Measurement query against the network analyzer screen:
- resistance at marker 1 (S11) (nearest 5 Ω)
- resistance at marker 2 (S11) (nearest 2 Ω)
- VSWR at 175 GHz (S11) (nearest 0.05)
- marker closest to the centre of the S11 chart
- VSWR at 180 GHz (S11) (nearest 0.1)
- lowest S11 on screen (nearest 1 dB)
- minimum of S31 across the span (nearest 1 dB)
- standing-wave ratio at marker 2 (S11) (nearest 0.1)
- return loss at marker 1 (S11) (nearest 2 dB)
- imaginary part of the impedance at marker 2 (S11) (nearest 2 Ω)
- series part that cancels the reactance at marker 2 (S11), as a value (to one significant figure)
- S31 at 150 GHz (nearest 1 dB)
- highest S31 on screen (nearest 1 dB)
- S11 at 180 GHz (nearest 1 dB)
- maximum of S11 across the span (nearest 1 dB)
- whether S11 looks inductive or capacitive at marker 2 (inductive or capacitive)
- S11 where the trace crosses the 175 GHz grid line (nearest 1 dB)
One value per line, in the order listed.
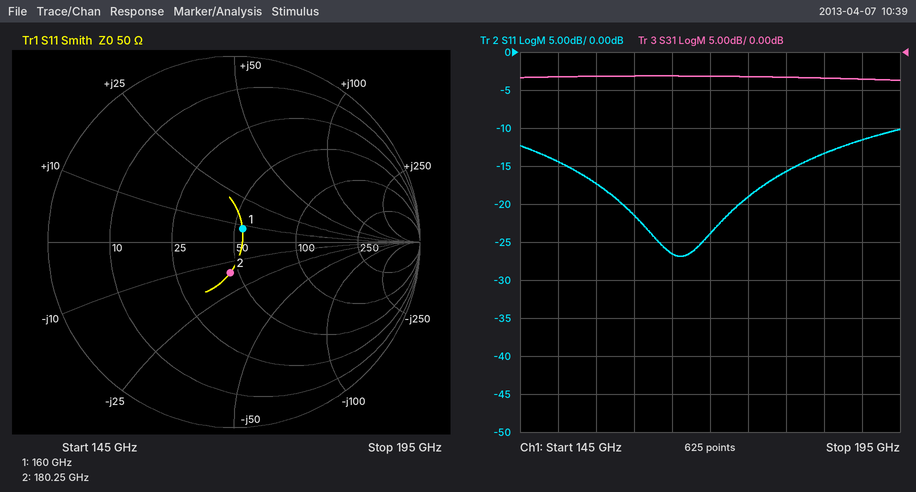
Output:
55 Ω
46 Ω
1.25
marker 1
1.4
-27 dB
-4 dB
1.4
22 dB
-16 Ω
10 pH
-3 dB
-3 dB
-16 dB
-10 dB
capacitive
-19 dB
